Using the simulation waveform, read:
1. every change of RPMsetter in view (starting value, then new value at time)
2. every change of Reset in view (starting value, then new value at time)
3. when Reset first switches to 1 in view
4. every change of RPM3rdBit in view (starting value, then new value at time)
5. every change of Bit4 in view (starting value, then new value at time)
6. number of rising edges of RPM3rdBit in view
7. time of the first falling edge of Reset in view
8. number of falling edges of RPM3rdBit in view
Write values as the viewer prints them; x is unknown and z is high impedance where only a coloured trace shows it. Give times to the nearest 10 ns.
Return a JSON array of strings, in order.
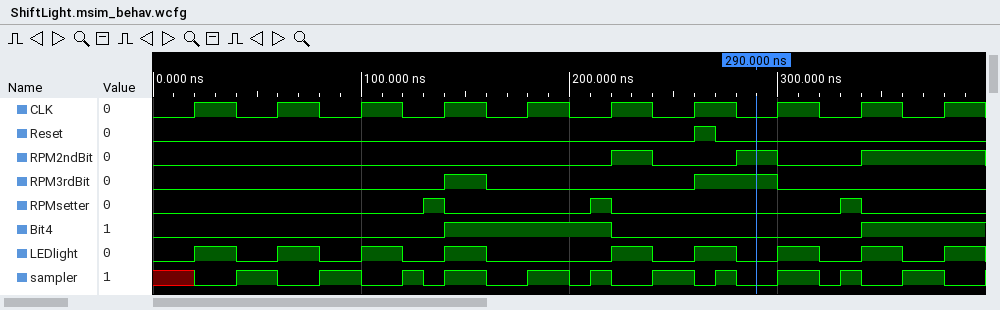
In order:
["0, 1 at 130 ns, 0 at 140 ns, 1 at 210 ns, 0 at 220 ns, 1 at 330 ns, 0 at 340 ns", "0, 1 at 260 ns, 0 at 270 ns", "260 ns", "0, 1 at 140 ns, 0 at 160 ns, 1 at 260 ns, 0 at 300 ns", "0, 1 at 140 ns, 0 at 220 ns, 1 at 340 ns", "2", "270 ns", "2"]
